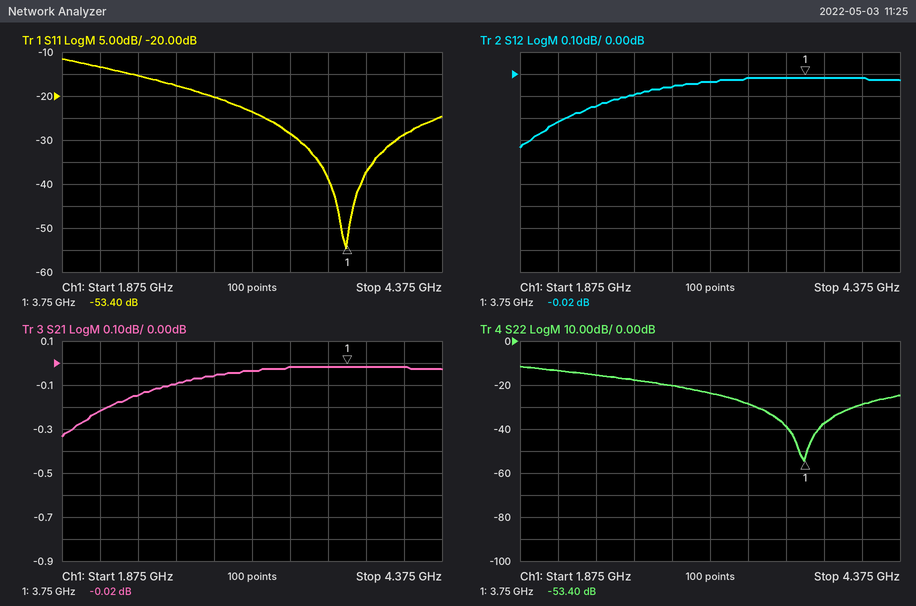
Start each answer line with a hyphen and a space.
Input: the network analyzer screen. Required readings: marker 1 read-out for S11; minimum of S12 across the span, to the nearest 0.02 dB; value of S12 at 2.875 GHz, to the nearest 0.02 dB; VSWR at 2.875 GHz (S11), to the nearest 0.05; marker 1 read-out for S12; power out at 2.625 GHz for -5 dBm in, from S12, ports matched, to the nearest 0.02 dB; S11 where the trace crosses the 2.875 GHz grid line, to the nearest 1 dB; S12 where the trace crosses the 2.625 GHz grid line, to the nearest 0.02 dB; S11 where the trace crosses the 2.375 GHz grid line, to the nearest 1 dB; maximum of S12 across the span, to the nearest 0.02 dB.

- -53.40 dB
- -0.34 dB
- -0.06 dB
- 1.20
- -0.02 dB
- -5.10 dBm
- -20 dB
- -0.10 dB
- -15 dB
- -0.02 dB
